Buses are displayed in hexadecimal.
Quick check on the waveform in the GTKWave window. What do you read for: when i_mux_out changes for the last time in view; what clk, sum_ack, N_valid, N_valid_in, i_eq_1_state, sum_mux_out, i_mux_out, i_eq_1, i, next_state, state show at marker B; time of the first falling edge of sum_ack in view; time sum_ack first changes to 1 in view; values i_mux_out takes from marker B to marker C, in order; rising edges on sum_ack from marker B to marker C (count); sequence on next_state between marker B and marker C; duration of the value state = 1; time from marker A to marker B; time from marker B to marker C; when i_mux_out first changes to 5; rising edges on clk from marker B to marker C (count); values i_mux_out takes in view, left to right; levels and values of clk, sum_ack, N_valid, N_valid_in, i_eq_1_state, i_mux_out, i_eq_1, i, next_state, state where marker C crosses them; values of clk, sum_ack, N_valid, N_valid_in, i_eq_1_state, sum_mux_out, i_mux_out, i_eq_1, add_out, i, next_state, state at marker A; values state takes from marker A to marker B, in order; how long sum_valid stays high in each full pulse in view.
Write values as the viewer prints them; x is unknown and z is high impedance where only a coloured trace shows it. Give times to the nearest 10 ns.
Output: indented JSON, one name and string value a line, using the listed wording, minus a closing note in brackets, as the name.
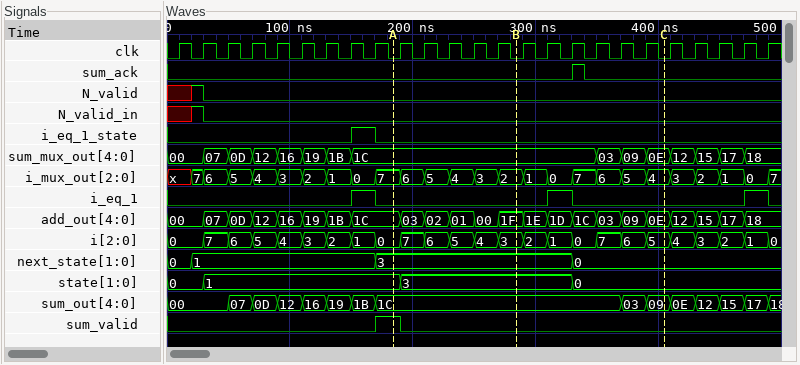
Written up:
{
  "when i_mux_out changes for the last time in view": "490 ns",
  "what clk, sum_ack, N_valid, N_valid_in, i_eq_1_state, sum_mux_out, i_mux_out, i_eq_1, i, next_state, state show at marker B": "clk=0, sum_ack=0, N_valid=0, N_valid_in=0, i_eq_1_state=0, sum_mux_out=1C, i_mux_out=2, i_eq_1=0, i=3, next_state=3, state=3",
  "time of the first falling edge of sum_ack in view": "340 ns",
  "time sum_ack first changes to 1 in view": "330 ns",
  "values i_mux_out takes from marker B to marker C, in order": "2, 1, 0, 7, 6, 5, 4",
  "rising edges on sum_ack from marker B to marker C": "1",
  "sequence on next_state between marker B and marker C": "3, 0",
  "duration of the value state = 1": "160 ns",
  "time from marker A to marker B": "100 ns",
  "time from marker B to marker C": "120 ns",
  "when i_mux_out first changes to 5": "50 ns",
  "rising edges on clk from marker B to marker C": "6",
  "values i_mux_out takes in view, left to right": "x, 7, 6, 5, 4, 3, 2, 1, 0, 7, 6, 5, 4, 3, 2, 1, 0, 7, 6, 5, 4, 3, 2, 1, 0, 7",
  "levels and values of clk, sum_ack, N_valid, N_valid_in, i_eq_1_state, i_mux_out, i_eq_1, i, next_state, state where marker C crosses them": "clk=0, sum_ack=0, N_valid=0, N_valid_in=0, i_eq_1_state=0, i_mux_out=4, i_eq_1=0, i=5, next_state=0, state=0",
  "values of clk, sum_ack, N_valid, N_valid_in, i_eq_1_state, sum_mux_out, i_mux_out, i_eq_1, add_out, i, next_state, state at marker A": "clk=0, sum_ack=0, N_valid=0, N_valid_in=0, i_eq_1_state=0, sum_mux_out=1C, i_mux_out=7, i_eq_1=0, add_out=1C, i=0, next_state=3, state=1",
  "values state takes from marker A to marker B, in order": "1, 3",
  "how long sum_valid stays high in each full pulse in view": "20 ns"
}
